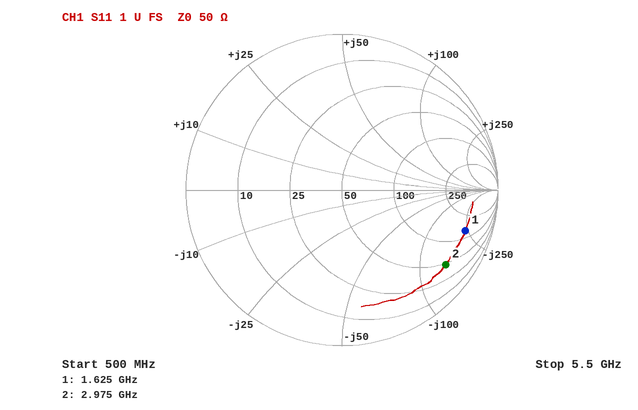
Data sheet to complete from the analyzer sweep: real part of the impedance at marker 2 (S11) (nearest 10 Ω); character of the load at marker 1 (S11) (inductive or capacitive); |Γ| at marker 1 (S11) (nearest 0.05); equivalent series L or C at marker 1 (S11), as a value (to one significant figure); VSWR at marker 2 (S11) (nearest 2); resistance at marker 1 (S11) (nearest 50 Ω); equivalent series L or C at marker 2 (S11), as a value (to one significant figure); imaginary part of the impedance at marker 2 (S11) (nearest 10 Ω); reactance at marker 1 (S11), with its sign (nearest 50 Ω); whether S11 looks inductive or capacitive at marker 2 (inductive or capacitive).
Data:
50 Ω
capacitive
0.85
400 fF
10
150 Ω
400 fF
-140 Ω
-250 Ω
capacitive
